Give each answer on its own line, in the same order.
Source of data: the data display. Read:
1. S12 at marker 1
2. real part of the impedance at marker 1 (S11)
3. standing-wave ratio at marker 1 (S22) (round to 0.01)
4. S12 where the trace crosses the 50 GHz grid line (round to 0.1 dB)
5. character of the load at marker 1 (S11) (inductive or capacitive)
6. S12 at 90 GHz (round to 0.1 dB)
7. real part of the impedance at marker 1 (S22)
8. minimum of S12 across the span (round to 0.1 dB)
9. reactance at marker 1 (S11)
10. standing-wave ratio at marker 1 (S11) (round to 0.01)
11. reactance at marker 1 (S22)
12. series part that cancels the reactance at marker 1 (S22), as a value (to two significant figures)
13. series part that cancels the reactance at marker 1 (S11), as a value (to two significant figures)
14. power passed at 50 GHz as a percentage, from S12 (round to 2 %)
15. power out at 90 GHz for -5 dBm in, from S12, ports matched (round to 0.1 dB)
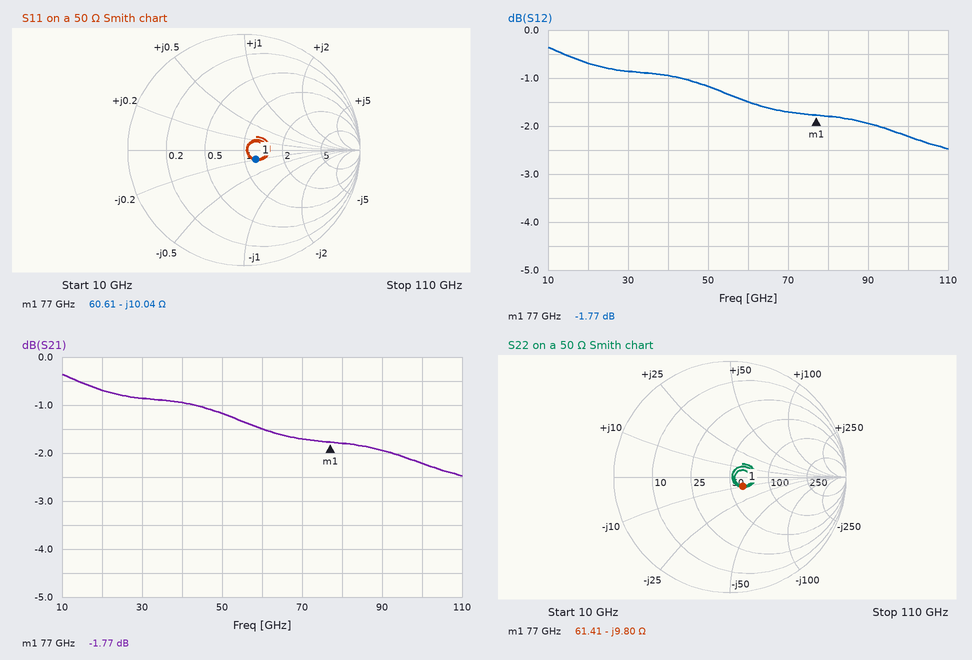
-1.77 dB
60.61 Ω
1.31
-1.2 dB
capacitive
-1.9 dB
61.41 Ω
-2.5 dB
-10.04 Ω
1.30
-9.80 Ω
20 pH
21 pH
76 %
-6.9 dBm
